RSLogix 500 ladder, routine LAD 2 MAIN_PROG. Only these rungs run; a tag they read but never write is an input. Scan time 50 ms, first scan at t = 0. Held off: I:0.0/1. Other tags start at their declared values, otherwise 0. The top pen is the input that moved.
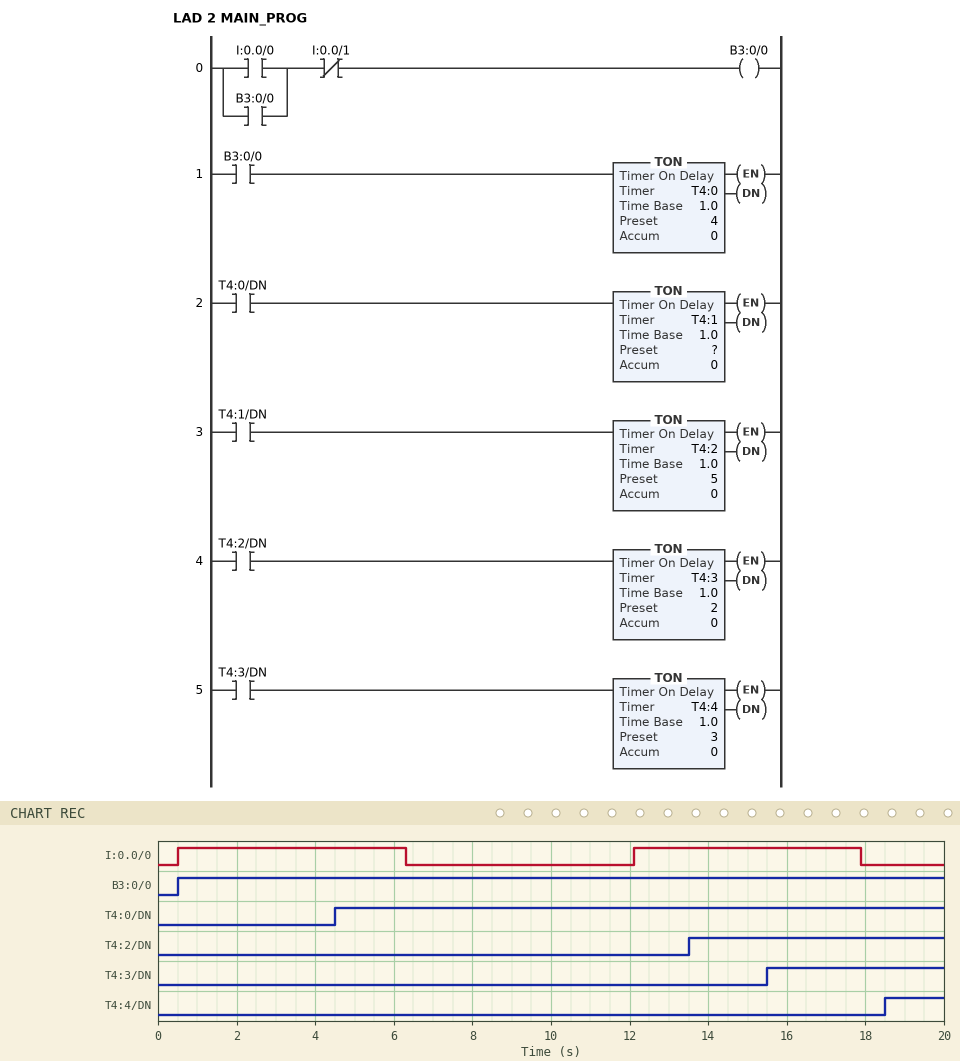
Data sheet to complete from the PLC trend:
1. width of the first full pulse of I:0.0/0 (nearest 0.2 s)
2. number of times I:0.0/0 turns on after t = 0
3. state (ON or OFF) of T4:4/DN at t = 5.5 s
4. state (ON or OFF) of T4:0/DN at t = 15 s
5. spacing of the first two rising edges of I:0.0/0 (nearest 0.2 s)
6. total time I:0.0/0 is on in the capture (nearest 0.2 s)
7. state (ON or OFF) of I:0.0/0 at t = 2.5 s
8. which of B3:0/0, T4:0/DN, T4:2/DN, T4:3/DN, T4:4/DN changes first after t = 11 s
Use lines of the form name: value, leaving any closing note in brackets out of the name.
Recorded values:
width of the first full pulse of I:0.0/0: 5.8 s
number of times I:0.0/0 turns on after t = 0: 2
state (ON or OFF) of T4:4/DN at t = 5.5 s: OFF
state (ON or OFF) of T4:0/DN at t = 15 s: ON
spacing of the first two rising edges of I:0.0/0: 11.6 s
total time I:0.0/0 is on in the capture: 11.6 s
state (ON or OFF) of I:0.0/0 at t = 2.5 s: ON
which of B3:0/0, T4:0/DN, T4:2/DN, T4:3/DN, T4:4/DN changes first after t = 11 s: T4:2/DN
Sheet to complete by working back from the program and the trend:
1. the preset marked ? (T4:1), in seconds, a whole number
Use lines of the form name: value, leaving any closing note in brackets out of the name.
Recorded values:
the preset marked ? (T4:1), in seconds, a whole number: 4 s
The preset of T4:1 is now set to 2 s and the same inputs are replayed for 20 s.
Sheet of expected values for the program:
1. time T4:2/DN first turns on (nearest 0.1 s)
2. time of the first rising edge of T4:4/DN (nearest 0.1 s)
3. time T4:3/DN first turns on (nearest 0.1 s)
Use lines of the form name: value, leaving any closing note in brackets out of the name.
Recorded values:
time T4:2/DN first turns on: 11.5 s
time of the first rising edge of T4:4/DN: 16.5 s
time T4:3/DN first turns on: 13.5 s
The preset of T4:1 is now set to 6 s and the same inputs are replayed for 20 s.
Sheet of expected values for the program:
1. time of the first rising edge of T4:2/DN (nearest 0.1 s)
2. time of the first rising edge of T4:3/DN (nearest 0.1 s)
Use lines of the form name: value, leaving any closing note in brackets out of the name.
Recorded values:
time of the first rising edge of T4:2/DN: 15.5 s
time of the first rising edge of T4:3/DN: 17.5 s
